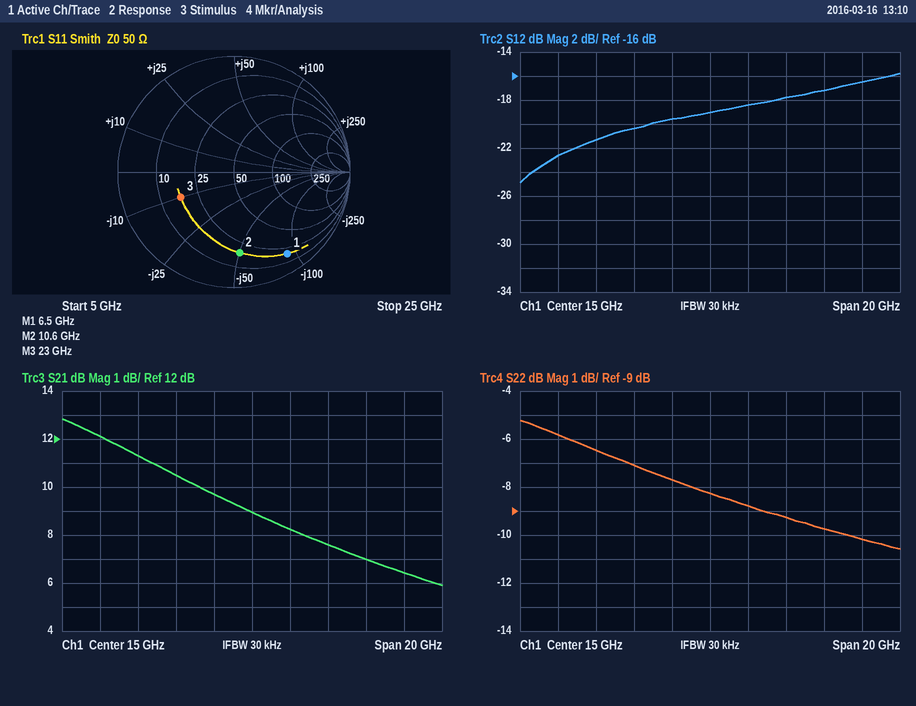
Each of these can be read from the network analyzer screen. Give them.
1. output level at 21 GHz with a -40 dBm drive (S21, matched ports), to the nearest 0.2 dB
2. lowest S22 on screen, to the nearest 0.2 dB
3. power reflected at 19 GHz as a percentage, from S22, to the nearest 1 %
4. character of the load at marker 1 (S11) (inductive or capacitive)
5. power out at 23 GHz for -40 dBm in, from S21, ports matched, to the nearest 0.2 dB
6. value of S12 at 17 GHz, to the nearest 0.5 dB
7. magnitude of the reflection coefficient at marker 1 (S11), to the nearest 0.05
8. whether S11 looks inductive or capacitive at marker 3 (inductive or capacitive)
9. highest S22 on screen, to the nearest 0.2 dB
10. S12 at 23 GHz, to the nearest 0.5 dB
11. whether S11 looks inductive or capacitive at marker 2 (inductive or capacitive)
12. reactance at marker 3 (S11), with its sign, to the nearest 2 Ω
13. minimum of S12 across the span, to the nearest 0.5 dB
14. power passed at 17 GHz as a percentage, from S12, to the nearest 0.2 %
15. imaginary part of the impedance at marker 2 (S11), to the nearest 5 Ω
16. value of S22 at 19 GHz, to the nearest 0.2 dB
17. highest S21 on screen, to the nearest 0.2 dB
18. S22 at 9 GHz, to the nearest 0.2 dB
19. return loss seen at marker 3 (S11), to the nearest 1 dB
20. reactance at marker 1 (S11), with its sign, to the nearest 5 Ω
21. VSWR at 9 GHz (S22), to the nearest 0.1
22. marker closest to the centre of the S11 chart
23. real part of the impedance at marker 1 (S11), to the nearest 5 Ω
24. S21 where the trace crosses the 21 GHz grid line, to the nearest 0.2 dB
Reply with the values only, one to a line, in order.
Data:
-33.0 dBm
-10.6 dB
12 %
capacitive
-33.6 dBm
-18.5 dB
0.85
capacitive
-5.2 dB
-16.5 dB
capacitive
-10 Ω
-25.0 dB
1.4 %
-50 Ω
-9.2 dB
12.8 dB
-6.4 dB
6 dB
-90 Ω
2.8
marker 3
20 Ω
7.0 dB
